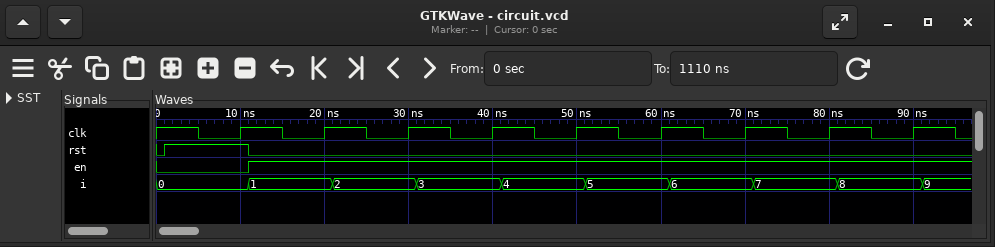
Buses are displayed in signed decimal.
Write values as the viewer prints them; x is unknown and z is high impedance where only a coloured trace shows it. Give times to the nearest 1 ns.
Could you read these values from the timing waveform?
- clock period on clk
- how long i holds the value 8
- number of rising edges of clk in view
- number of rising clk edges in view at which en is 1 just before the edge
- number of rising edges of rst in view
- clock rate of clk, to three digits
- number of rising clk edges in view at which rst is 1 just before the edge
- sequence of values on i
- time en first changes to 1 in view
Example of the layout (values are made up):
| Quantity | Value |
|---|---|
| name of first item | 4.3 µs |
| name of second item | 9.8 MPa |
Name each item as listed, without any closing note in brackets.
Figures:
| Quantity | Value |
|---|---|
| clock period on clk | 10 ns |
| how long i holds the value 8 | 10 ns |
| number of rising edges of clk in view | 9 |
| number of rising clk edges in view at which en is 1 just before the edge | 8 |
| number of rising edges of rst in view | 1 |
| clock rate of clk, to three digits | 100 MHz |
| number of rising clk edges in view at which rst is 1 just before the edge | 1 |
| sequence of values on i | 0, 1, 2, 3, 4, 5, 6, 7, 8, 9 |
| time en first changes to 1 in view | 11 ns |
